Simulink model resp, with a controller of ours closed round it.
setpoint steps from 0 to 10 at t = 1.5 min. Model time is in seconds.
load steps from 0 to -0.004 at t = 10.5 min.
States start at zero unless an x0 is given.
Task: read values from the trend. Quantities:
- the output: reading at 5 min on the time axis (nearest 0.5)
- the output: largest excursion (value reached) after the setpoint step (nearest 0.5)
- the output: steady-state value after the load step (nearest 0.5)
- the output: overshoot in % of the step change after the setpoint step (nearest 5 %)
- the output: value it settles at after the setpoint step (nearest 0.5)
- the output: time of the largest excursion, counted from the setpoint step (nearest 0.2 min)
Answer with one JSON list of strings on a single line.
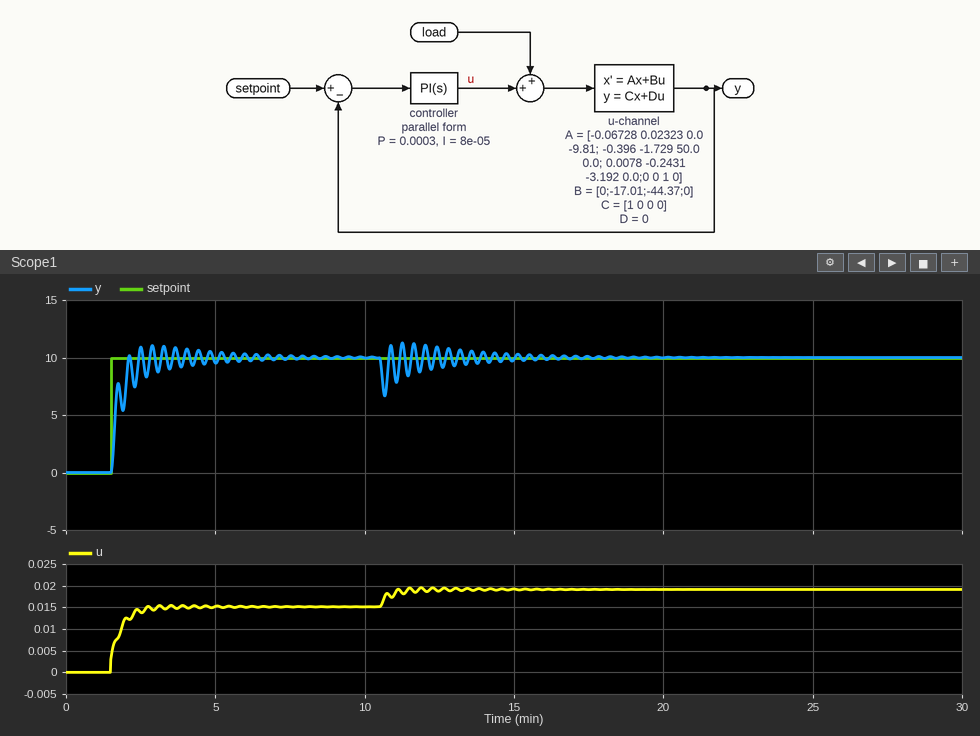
["9.5", "11.0", "10.0", "10 %", "10.0", "1.4 min"]
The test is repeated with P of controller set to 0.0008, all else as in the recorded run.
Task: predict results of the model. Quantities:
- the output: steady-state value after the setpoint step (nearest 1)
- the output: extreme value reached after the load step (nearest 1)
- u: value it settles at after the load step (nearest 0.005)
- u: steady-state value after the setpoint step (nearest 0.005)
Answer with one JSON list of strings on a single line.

["10", "7", "0.020", "0.015"]
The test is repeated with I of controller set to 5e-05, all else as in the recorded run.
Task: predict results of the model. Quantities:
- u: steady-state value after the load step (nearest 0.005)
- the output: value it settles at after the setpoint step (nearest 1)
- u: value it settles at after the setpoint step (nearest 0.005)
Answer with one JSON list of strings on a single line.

["0.020", "10", "0.015"]
